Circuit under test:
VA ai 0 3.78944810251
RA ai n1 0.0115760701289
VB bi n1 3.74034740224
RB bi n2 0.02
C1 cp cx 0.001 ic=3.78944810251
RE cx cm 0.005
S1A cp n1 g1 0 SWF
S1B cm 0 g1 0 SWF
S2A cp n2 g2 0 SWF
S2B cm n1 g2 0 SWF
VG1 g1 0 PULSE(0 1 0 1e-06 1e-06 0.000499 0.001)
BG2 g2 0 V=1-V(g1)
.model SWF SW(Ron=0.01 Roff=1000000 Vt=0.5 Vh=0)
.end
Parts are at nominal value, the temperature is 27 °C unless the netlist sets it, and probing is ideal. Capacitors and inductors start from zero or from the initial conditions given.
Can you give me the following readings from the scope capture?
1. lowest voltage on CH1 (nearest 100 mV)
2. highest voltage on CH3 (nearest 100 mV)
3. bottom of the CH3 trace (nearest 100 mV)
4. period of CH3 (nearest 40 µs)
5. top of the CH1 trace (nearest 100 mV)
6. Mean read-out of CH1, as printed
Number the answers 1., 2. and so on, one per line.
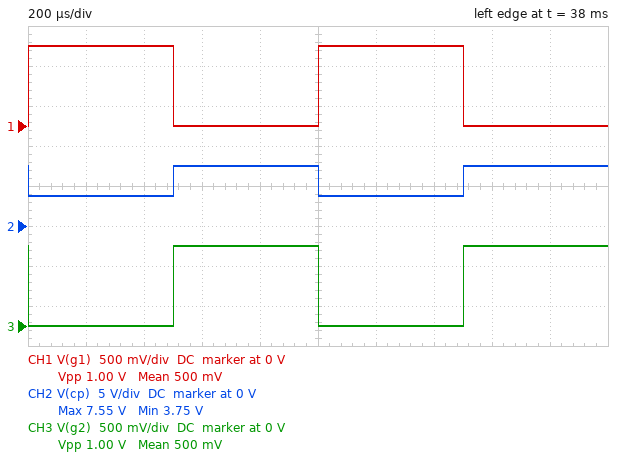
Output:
1. 0 V
2. 1.0 V
3. 0 V
4. 1.00 ms
5. 1.0 V
6. 500 mV
